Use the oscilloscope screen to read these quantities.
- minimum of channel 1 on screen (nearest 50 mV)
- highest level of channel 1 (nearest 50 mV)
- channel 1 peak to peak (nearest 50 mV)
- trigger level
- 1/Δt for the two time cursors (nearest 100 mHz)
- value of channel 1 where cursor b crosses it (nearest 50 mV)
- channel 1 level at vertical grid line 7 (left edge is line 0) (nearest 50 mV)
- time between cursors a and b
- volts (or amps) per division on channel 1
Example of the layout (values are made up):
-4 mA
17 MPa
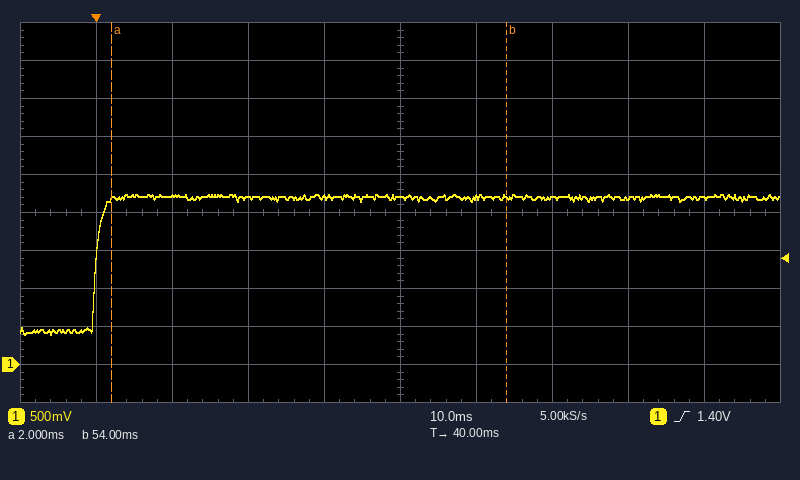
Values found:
400 mV
2.25 V
1.85 V
1.40 V
19.2 Hz
2.20 V
2.20 V
52 ms
500 mV
